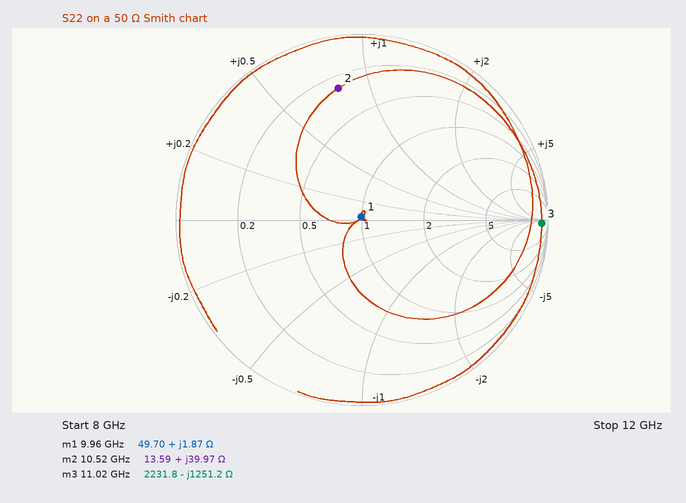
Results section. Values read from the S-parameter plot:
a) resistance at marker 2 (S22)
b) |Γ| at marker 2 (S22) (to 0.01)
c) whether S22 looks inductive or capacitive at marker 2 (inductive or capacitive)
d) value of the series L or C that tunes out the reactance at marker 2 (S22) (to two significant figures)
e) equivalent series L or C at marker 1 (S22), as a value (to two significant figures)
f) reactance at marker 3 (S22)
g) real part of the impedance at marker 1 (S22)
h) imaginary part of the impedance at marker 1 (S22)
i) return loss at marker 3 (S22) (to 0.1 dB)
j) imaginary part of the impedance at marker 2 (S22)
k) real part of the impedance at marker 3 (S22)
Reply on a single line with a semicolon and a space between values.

13.59 Ω; 0.72; inductive; 380 fF; 30 pH; -1251.2 Ω; 49.70 Ω; +1.87 Ω; 0.3 dB; +39.97 Ω; 2231.8 Ω
